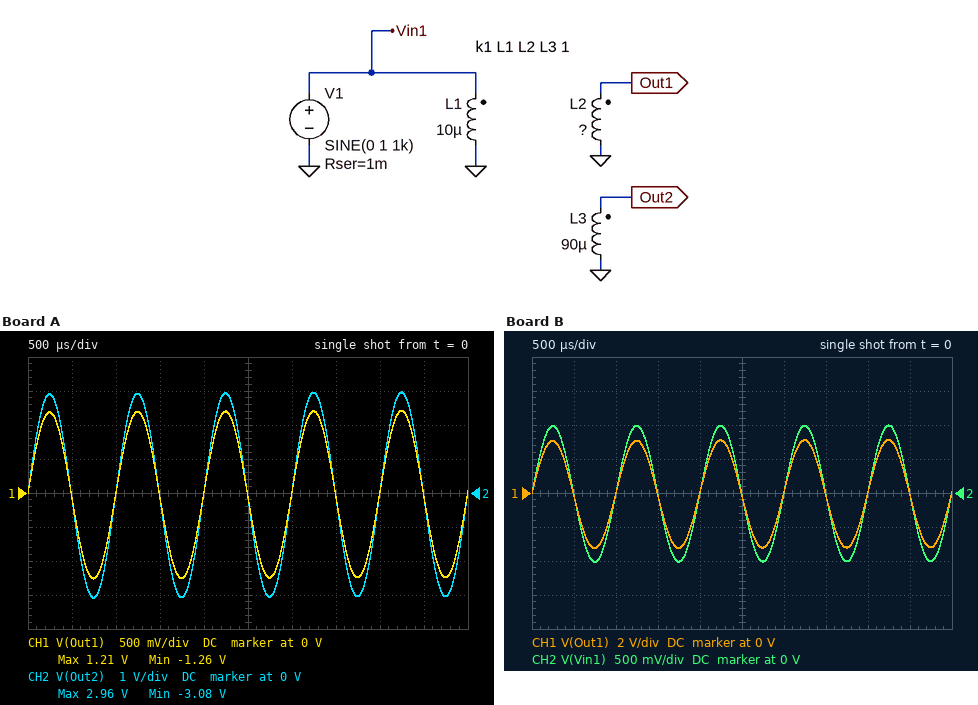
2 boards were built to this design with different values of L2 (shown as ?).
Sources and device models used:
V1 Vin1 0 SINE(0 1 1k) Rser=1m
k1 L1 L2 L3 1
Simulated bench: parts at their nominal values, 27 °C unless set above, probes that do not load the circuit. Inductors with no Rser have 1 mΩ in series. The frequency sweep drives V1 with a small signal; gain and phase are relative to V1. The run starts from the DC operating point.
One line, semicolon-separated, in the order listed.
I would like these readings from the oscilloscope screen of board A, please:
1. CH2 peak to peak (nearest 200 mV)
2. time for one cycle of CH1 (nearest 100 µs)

6.0 V; 1.0 ms
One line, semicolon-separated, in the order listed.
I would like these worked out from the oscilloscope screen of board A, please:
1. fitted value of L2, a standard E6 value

15 µH
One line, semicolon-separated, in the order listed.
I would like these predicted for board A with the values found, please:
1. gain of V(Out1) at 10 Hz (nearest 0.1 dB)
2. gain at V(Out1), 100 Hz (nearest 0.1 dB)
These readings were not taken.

-8.7 dB; 1.3 dB
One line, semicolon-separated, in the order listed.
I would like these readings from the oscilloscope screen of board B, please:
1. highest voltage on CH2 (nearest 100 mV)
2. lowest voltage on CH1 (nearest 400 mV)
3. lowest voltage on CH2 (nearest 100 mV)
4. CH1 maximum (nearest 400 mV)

1.0 V; -3.2 V; -1.0 V; 3.2 V
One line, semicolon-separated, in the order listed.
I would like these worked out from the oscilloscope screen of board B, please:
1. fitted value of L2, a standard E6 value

100 µH
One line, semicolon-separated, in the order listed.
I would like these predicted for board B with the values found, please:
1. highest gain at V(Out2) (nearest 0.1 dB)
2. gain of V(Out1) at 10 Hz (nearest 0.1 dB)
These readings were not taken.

9.5 dB; -0.5 dB
